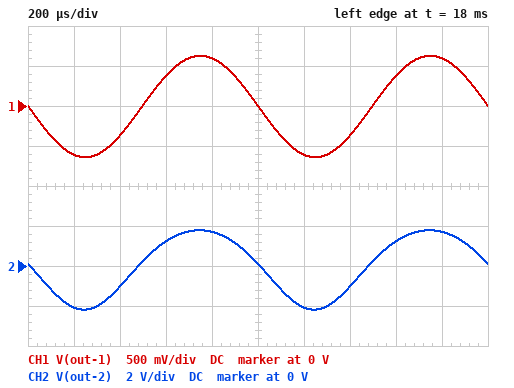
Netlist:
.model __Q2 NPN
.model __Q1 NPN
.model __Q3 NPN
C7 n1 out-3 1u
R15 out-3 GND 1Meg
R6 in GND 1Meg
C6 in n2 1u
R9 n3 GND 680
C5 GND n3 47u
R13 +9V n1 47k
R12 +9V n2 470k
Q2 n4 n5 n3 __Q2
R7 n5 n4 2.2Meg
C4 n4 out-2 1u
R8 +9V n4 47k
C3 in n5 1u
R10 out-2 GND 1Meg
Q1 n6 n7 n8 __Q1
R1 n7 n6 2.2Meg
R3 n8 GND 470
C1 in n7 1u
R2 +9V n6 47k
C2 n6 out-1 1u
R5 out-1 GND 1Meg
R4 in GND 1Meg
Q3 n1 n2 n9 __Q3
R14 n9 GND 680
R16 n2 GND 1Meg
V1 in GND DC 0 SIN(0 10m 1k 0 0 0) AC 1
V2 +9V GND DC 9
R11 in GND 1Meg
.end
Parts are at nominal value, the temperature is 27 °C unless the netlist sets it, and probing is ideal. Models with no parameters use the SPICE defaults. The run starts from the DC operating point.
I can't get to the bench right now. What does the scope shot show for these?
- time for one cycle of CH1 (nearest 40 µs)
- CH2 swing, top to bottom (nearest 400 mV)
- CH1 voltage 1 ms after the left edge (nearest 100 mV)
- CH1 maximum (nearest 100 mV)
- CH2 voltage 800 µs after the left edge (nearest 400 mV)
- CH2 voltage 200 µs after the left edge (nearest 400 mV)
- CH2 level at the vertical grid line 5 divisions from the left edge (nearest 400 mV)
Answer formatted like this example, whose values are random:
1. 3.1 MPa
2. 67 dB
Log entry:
1. 1.00 ms
2. 4.0 V
3. 0 V
4. 600 mV
5. 1.6 V
6. -2.0 V
7. 0 V
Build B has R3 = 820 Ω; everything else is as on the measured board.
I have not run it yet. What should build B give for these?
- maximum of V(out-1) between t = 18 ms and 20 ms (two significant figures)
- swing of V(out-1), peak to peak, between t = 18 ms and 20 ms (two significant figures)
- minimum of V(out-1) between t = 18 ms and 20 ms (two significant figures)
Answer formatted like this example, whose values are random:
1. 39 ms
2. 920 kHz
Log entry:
1. 420 mV
2. 840 mV
3. -420 mV
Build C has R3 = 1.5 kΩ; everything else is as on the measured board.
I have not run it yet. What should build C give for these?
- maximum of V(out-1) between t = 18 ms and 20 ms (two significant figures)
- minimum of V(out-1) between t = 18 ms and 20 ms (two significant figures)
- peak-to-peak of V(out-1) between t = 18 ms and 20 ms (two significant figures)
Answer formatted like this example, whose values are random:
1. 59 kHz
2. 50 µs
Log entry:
1. 250 mV
2. -250 mV
3. 510 mV
